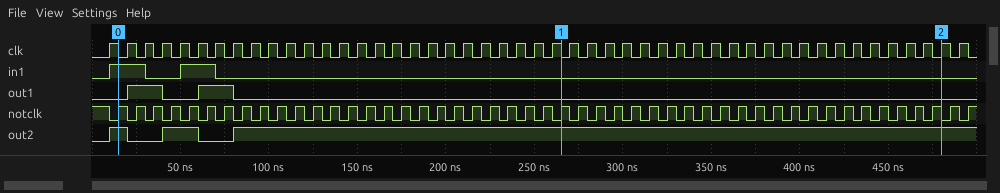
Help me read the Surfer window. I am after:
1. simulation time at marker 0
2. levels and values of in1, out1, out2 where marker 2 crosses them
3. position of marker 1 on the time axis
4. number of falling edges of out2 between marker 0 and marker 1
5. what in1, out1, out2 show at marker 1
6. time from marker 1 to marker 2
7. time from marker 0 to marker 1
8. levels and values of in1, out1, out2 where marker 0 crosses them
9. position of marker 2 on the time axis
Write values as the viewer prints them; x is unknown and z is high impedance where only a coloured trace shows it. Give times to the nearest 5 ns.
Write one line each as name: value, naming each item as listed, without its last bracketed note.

simulation time at marker 0: 15 ns
levels and values of in1, out1, out2 where marker 2 crosses them: in1=0, out1=0, out2=1
position of marker 1 on the time axis: 265 ns
number of falling edges of out2 between marker 0 and marker 1: 2
what in1, out1, out2 show at marker 1: in1=0, out1=0, out2=1
time from marker 1 to marker 2: 215 ns
time from marker 0 to marker 1: 250 ns
levels and values of in1, out1, out2 where marker 0 crosses them: in1=1, out1=0, out2=1
position of marker 2 on the time axis: 480 ns
